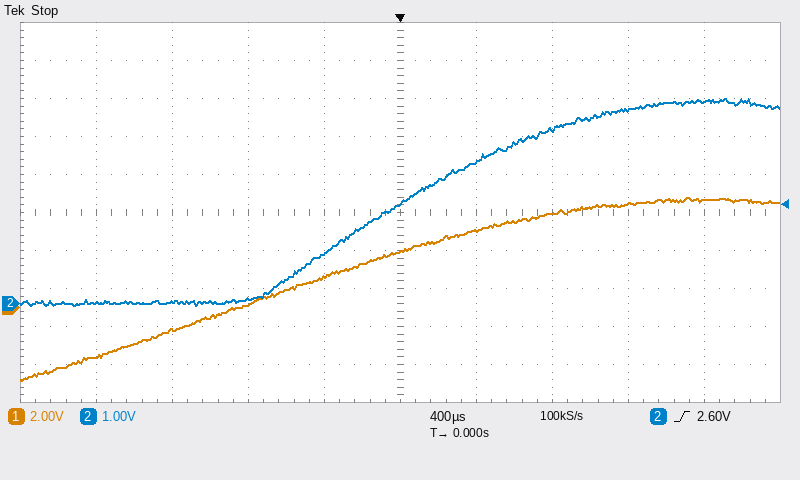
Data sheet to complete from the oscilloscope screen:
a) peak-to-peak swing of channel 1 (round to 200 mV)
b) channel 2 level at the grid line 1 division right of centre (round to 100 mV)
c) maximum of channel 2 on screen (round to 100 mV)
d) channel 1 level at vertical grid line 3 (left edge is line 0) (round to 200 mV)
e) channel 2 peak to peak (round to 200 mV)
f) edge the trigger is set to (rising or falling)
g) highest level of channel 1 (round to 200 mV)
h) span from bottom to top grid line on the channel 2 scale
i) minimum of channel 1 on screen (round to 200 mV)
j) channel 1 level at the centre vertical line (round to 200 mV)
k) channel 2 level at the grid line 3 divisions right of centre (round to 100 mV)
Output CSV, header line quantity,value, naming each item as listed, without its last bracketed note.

quantity,value
peak-to-peak swing of channel 1,9.6 V
channel 2 level at the grid line 1 division right of centre,3.7 V
maximum of channel 2 on screen,5.4 V
channel 1 level at vertical grid line 3 (left edge is line 0),200 mV
channel 2 peak to peak,5.4 V
edge the trigger is set to,rising
highest level of channel 1,5.8 V
span from bottom to top grid line on the channel 2 scale,10 V
minimum of channel 1 on screen,-3.8 V
channel 1 level at the centre vertical line,3.0 V
channel 2 level at the grid line 3 divisions right of centre,5.1 V
